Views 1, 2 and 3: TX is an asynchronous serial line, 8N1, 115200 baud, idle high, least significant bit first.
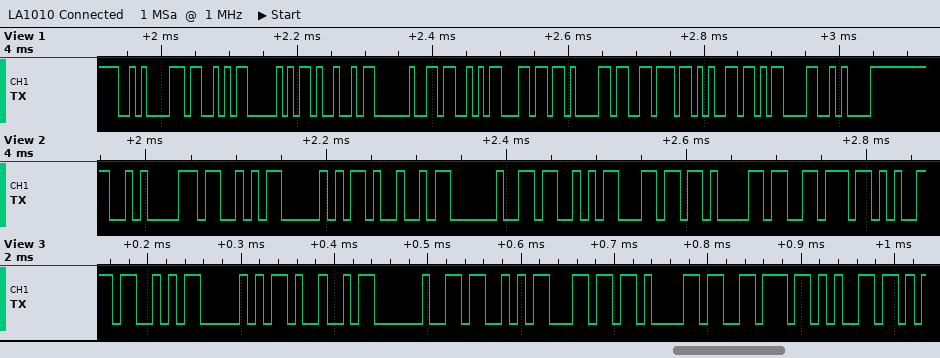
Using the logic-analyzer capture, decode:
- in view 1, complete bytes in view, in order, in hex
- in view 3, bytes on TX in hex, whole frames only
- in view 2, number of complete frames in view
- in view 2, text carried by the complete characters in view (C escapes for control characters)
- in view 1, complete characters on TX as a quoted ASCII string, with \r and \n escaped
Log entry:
0A 53 50 49 20 53 6C 61 76 65 0D 0A
53 50 49 20 53 6C 61 76 65
9
"\nSPI Slav"
"\nSPI Slave\r\n"
